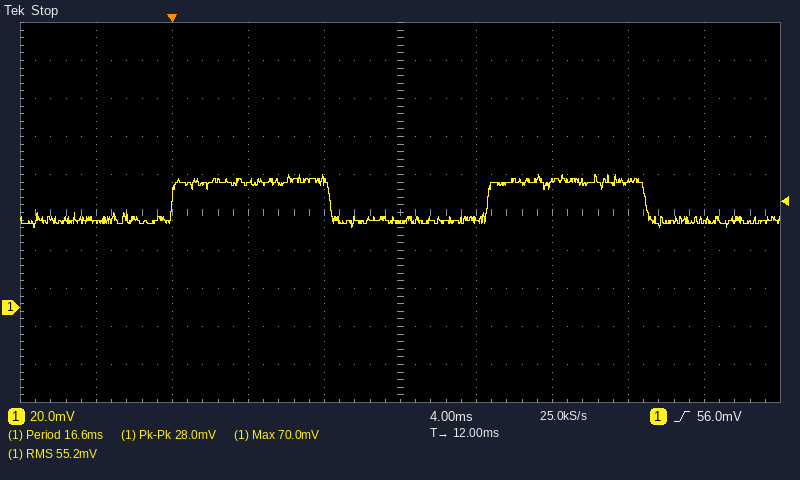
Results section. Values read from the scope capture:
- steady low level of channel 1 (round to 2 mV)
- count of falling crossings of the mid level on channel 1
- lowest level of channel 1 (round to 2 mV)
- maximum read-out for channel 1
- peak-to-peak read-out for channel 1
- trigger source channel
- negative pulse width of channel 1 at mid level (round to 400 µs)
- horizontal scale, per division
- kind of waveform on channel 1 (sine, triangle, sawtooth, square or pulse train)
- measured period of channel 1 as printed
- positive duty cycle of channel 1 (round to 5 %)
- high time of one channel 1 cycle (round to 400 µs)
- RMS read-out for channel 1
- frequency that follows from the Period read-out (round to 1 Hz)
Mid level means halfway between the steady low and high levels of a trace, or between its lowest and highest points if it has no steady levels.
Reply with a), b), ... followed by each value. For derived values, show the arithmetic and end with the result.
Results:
a) 46 mV
b) 2
c) 42 mV
d) 70.0 mV
e) 28.0 mV
f) channel 1
g) 8.4 ms
h) 4 ms
i) square
j) 16.6 ms
k) 50 %
l) 8.4 ms
m) 55.2 mV
n) 1 / 16.6 ms ≈ 60 Hz
